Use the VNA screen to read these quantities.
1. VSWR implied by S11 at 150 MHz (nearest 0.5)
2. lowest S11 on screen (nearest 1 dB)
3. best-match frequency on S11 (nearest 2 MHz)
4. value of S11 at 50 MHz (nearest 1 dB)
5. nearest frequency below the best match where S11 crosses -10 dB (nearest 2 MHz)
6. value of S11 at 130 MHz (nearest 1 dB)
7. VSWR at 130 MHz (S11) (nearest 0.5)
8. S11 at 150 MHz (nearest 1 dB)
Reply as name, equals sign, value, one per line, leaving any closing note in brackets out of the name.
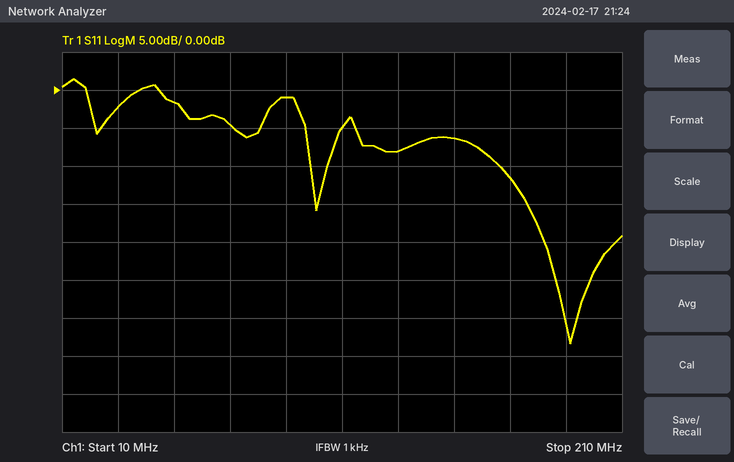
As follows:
VSWR implied by S11 at 150 MHz = 3.0
lowest S11 on screen = -33 dB
best-match frequency on S11 = 192 MHz
value of S11 at 50 MHz = -2 dB
nearest frequency below the best match where S11 crosses -10 dB = 166 MHz
value of S11 at 130 MHz = -8 dB
VSWR at 130 MHz (S11) = 2.5
S11 at 150 MHz = -6 dB
